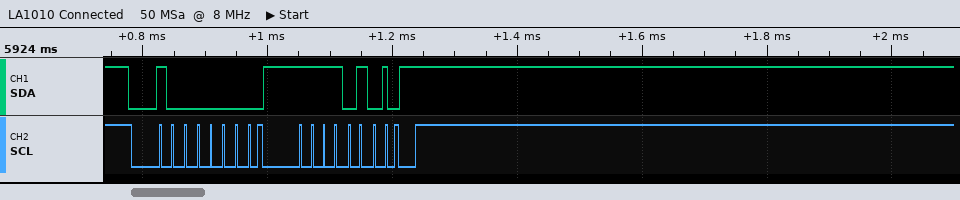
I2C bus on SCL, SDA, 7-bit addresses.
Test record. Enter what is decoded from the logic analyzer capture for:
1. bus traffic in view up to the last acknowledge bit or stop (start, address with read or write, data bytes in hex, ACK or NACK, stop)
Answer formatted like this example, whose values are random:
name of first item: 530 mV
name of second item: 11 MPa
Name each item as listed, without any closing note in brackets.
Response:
bus traffic in view up to the last acknowledge bit or stop: start, address 40 write ACK, F5 ACK
